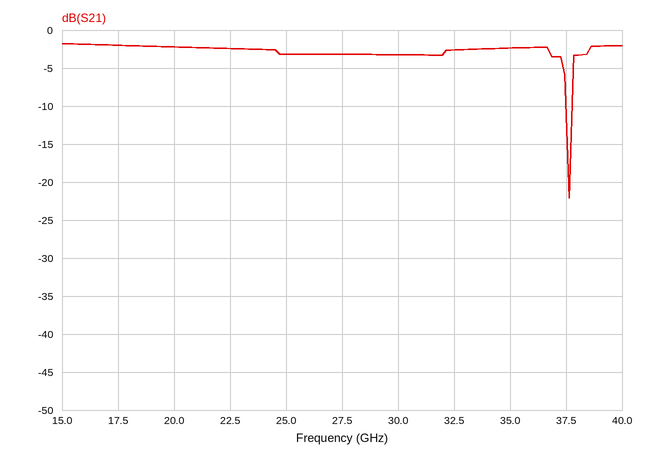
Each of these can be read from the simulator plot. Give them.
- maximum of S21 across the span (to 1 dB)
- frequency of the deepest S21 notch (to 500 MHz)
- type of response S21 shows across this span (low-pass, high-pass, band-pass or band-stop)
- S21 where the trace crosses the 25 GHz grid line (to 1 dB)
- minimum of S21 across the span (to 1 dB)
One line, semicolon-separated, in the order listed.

-2 dB; 37.5 GHz; band-stop; -3 dB; -22 dB
